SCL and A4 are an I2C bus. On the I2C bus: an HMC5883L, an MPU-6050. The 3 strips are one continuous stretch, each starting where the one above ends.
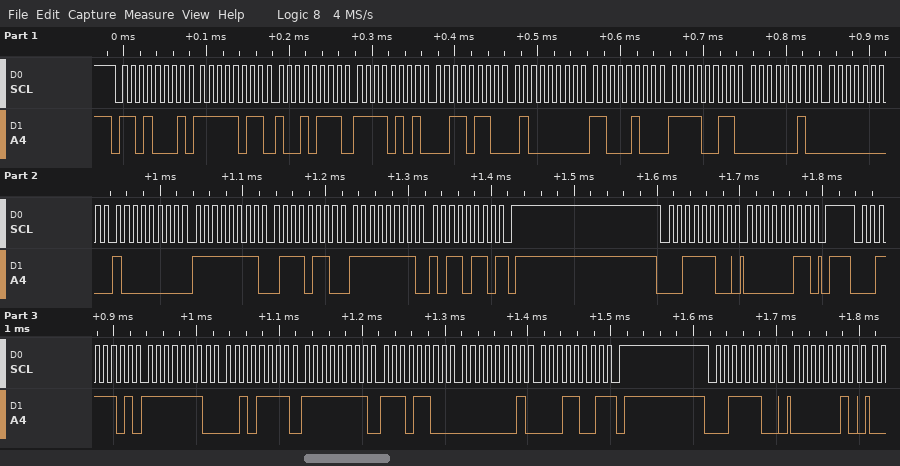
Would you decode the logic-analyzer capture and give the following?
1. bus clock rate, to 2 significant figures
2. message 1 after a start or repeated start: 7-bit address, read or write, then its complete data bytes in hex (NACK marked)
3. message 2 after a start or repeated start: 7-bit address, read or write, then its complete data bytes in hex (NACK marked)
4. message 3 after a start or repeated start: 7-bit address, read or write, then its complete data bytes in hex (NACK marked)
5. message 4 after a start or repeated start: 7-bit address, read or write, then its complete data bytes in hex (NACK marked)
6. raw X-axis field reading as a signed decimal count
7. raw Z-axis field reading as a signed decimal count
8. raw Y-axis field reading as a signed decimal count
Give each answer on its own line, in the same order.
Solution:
100 kHz
0x68 read: FB 97 F5 36 40 C4 F3 02 00 80 FF 76 FF B6 NACK
0x1E write: 03
0x1E read: FE 2F FF EC 01 19 NACK
0x1E write: 02
-465
-20
281
